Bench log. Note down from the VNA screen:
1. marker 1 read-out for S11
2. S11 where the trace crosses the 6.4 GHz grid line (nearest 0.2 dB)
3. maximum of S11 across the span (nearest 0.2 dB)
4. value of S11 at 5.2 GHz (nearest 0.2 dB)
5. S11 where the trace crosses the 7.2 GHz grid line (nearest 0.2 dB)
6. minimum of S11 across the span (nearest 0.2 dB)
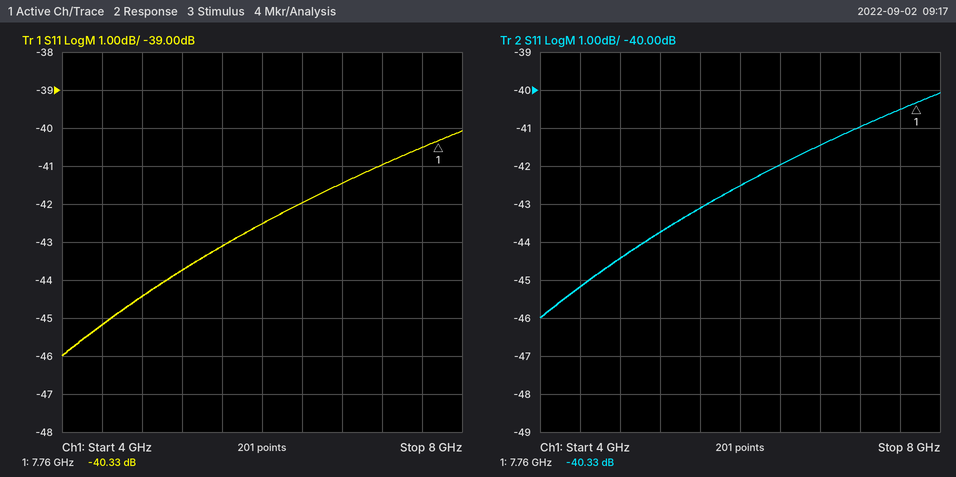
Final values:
-40.33 dB
-42.0 dB
-40.0 dB
-43.8 dB
-41.0 dB
-46.0 dB
